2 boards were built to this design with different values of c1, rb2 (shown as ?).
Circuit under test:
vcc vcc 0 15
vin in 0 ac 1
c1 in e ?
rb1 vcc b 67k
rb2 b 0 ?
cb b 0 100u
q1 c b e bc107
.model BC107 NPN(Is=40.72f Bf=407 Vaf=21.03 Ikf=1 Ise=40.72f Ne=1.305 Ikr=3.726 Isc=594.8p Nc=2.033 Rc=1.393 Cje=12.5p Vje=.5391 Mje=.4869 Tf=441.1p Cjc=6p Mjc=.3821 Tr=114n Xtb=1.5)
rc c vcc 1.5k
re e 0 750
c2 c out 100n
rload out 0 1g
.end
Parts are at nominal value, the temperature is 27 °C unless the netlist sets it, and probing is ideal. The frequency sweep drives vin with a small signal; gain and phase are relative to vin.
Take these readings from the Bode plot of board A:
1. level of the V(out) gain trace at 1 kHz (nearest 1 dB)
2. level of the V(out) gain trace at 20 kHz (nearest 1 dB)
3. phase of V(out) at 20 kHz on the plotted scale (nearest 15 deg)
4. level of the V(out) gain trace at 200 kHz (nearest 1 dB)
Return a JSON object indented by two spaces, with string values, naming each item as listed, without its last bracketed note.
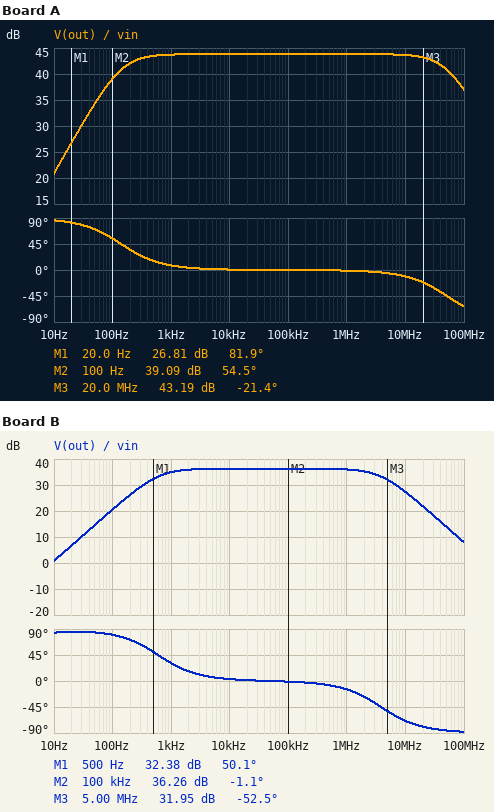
{
  "level of the V(out) gain trace at 1 kHz": "44 dB",
  "level of the V(out) gain trace at 20 kHz": "44 dB",
  "phase of V(out) at 20 kHz on the plotted scale": "0 deg",
  "level of the V(out) gain trace at 200 kHz": "44 dB"
}
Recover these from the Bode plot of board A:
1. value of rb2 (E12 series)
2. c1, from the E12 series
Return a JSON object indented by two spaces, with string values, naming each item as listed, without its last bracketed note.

{
  "value of rb2": "18 kΩ",
  "c1, from the E12 series": "120 µF"
}
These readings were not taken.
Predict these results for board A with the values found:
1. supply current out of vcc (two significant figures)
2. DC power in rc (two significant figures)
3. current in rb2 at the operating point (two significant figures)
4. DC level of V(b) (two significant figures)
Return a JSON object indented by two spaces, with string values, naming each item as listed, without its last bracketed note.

{
  "supply current out of vcc": "3.3 mA",
  "DC power in rc": "15 mW",
  "current in rb2 at the operating point": "170 µA",
  "DC level of V(b)": "3.0 V"
}
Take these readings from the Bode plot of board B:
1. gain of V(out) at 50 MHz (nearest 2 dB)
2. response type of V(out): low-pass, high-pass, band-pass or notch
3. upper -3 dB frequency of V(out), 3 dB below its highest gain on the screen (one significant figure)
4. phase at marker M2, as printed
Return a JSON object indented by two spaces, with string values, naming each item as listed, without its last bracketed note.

{
  "gain of V(out) at 50 MHz": "14 dB",
  "response type of V(out): low-pass, high-pass, band-pass or notch": "band-pass",
  "upper -3 dB frequency of V(out), 3 dB below its highest gain on the screen": "4 MHz",
  "phase at marker M2, as printed": "-1.1 deg"
}
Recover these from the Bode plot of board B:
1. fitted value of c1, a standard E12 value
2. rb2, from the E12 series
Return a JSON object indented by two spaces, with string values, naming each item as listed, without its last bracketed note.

{
  "fitted value of c1, a standard E12 value": "56 µF",
  "rb2, from the E12 series": "100 kΩ"
}
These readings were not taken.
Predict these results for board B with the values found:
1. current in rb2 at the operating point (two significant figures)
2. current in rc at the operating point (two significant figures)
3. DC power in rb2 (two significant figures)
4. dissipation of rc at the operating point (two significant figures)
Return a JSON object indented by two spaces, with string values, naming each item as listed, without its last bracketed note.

{
  "current in rb2 at the operating point": "57 µA",
  "current in rc at the operating point": "6.6 mA",
  "DC power in rb2": "320 µW",
  "dissipation of rc at the operating point": "65 mW"
}
